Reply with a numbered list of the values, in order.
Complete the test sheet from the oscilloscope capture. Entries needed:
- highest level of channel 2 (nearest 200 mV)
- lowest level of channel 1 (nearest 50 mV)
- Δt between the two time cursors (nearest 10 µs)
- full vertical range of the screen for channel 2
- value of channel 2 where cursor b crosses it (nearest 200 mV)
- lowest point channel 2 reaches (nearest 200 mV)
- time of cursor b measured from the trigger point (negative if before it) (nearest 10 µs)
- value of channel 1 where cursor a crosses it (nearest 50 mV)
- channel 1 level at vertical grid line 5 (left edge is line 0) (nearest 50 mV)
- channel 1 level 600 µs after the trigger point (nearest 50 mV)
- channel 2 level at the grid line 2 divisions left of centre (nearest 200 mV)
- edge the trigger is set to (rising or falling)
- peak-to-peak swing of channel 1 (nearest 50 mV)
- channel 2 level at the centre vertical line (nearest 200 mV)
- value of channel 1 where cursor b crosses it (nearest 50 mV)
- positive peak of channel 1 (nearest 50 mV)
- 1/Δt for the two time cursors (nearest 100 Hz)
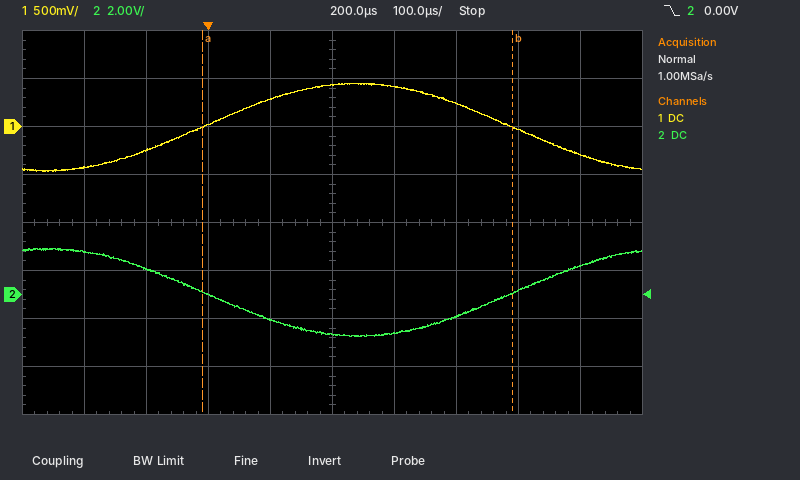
1. 2.0 V
2. -450 mV
3. 500 µs
4. 16 V
5. 0.0 V
6. -1.8 V
7. +490 µs
8. 0 mV
9. 450 mV
10. -300 mV
11. 0.0 V
12. falling
13. 900 mV
14. -1.6 V
15. 0 mV
16. 450 mV
17. 2.0 kHz
